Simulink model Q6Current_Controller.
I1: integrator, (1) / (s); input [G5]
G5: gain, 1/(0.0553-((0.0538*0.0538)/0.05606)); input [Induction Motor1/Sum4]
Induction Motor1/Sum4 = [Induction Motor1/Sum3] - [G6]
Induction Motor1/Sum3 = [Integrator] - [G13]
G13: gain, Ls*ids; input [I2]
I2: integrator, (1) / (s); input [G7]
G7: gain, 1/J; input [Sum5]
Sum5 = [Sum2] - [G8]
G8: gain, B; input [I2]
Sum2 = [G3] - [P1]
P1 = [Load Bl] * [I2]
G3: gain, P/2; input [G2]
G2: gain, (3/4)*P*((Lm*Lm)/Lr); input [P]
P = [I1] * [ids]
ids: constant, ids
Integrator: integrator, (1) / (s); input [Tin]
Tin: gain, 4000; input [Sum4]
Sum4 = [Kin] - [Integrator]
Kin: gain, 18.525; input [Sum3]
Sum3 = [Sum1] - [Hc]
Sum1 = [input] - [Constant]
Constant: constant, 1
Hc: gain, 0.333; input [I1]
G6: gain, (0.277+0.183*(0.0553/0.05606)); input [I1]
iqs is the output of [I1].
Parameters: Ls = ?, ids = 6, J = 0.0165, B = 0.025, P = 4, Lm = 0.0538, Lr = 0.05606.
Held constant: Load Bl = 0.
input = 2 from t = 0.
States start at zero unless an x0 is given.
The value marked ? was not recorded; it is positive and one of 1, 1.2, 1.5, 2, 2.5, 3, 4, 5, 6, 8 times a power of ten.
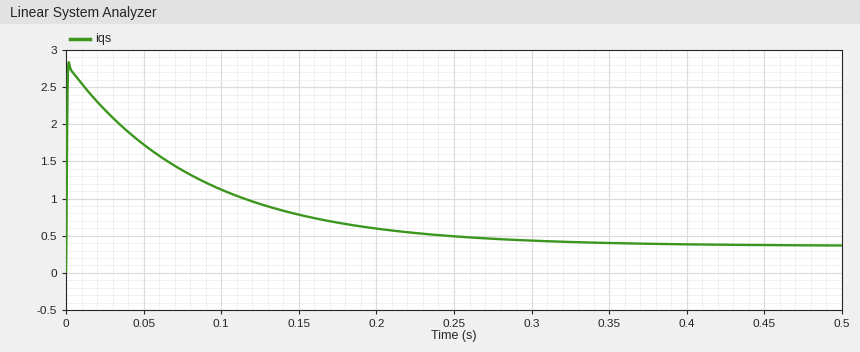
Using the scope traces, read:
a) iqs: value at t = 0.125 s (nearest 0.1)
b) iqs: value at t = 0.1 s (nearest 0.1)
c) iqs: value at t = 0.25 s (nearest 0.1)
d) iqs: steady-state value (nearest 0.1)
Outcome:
0.9
1.1
0.5
0.4
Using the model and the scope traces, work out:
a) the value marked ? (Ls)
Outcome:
0.1
